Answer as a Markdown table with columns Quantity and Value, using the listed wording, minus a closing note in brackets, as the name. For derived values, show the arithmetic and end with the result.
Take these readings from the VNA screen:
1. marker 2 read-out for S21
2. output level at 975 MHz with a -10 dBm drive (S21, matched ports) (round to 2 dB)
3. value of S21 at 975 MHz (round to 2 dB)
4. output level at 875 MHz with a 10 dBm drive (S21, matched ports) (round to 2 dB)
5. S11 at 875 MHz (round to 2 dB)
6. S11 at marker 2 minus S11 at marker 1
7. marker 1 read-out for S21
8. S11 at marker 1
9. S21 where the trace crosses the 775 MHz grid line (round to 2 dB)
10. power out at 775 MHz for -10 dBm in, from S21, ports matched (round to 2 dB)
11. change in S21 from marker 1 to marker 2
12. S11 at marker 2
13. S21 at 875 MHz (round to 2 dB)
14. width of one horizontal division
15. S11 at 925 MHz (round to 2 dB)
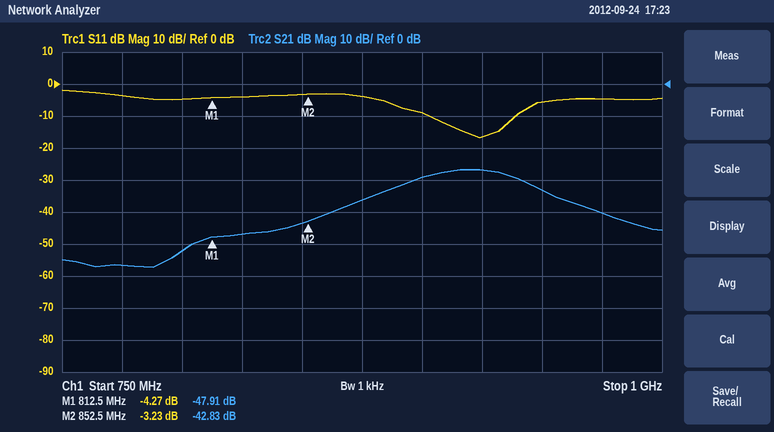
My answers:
| Quantity | Value |
|---|---|
| marker 2 read-out for S21 | -42.83 dB |
| output level at 975 MHz with a -10 dBm drive (S21, matched ports) | -10 dBm + (-40 dB) = -50 dBm |
| value of S21 at 975 MHz | -40 dB |
| output level at 875 MHz with a 10 dBm drive (S21, matched ports) | 10 dBm + (-36 dB) = -26 dBm |
| S11 at 875 MHz | -4 dB |
| S11 at marker 2 minus S11 at marker 1 | -3.23 − (-4.27) = 1.04 dB |
| marker 1 read-out for S21 | -47.91 dB |
| S11 at marker 1 | -4.27 dB |
| S21 where the trace crosses the 775 MHz grid line | -56 dB |
| power out at 775 MHz for -10 dBm in, from S21, ports matched | -10 dBm + (-56 dB) = -66 dBm |
| change in S21 from marker 1 to marker 2 | -42.83 − (-47.91) = 5.08 dB |
| S11 at marker 2 | -3.23 dB |
| S21 at 875 MHz | -36 dB |
| width of one horizontal division | 25 MHz |
| S11 at 925 MHz | -16 dB |
